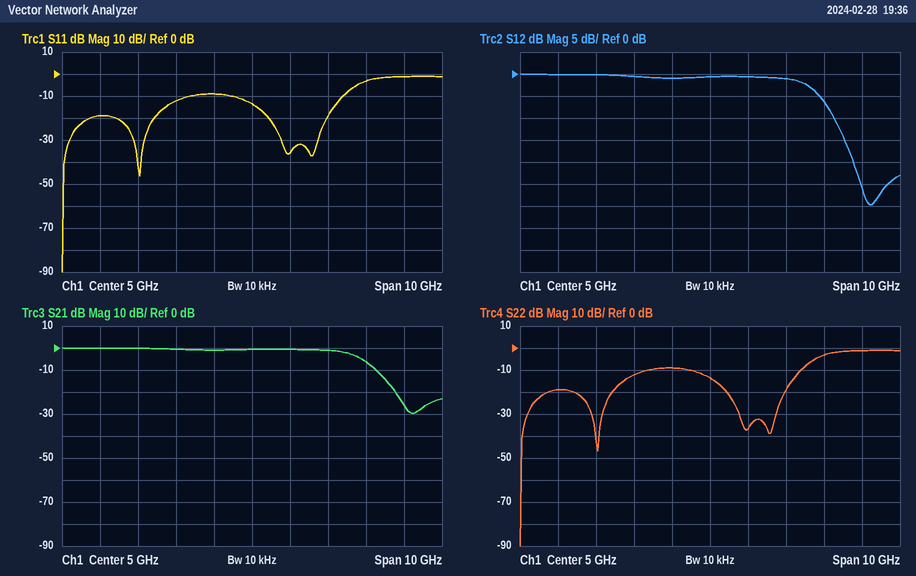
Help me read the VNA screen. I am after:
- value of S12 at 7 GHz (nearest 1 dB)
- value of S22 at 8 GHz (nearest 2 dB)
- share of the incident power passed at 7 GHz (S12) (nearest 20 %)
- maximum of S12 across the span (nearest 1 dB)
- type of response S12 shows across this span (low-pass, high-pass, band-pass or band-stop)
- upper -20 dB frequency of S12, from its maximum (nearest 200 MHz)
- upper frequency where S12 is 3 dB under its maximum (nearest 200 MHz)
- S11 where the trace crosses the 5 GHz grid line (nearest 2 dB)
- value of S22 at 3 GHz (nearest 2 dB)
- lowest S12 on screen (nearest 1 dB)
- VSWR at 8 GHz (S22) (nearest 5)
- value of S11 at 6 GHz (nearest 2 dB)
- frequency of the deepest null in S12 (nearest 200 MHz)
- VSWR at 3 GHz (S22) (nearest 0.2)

-1 dB
-4 dB
80 %
0 dB
low-pass
8.8 GHz
7.6 GHz
-14 dB
-12 dB
-30 dB
5
-36 dB
9.2 GHz
1.6
